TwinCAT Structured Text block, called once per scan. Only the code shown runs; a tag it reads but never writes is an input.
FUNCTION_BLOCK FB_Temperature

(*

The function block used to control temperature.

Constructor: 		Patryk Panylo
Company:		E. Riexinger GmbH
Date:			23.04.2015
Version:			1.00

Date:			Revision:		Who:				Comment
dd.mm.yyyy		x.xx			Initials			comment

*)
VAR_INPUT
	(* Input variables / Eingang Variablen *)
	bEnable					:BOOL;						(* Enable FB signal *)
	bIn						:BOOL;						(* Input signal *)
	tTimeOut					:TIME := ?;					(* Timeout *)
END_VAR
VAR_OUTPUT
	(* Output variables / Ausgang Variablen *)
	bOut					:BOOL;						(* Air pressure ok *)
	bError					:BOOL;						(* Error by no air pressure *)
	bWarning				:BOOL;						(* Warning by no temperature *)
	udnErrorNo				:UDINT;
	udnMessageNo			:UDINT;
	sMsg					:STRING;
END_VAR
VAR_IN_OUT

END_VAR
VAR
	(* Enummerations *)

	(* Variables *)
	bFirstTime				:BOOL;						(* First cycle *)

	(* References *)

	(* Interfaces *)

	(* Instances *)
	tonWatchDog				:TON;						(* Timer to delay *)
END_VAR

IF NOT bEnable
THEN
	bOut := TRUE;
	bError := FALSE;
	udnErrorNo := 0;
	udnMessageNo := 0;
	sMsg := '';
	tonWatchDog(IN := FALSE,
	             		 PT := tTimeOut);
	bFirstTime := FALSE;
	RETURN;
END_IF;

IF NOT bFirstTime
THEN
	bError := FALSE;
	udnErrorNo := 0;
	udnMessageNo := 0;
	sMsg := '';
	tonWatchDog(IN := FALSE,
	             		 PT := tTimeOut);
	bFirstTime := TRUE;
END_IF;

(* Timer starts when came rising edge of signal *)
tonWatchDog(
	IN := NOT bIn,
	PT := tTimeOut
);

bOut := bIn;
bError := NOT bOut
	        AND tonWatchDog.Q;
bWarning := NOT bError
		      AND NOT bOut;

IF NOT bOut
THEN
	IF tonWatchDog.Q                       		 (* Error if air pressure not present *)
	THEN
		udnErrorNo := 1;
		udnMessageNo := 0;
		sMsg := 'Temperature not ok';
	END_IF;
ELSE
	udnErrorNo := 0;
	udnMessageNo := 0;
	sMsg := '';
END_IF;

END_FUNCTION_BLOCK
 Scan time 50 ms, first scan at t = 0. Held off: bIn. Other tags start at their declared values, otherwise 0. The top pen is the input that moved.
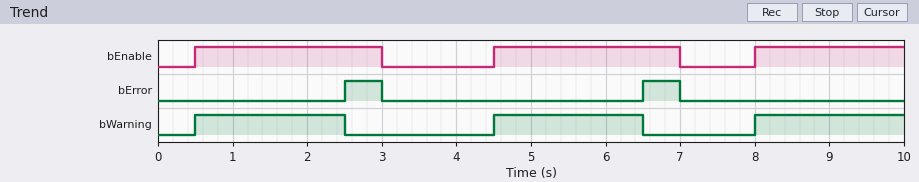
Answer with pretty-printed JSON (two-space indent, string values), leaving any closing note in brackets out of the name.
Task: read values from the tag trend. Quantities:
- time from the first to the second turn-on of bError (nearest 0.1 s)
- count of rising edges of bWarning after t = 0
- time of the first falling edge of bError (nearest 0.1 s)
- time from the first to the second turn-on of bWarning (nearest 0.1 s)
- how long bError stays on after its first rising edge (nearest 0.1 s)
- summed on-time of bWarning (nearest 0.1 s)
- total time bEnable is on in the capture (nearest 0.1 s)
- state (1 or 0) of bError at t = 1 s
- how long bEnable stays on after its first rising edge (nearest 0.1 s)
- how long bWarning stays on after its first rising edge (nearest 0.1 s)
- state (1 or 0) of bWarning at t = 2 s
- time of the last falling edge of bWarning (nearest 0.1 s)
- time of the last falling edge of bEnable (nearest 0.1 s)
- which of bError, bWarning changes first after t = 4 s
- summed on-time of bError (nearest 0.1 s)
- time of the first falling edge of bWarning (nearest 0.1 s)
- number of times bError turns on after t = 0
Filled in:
{
  "time from the first to the second turn-on of bError": "4.0 s",
  "count of rising edges of bWarning after t = 0": "3",
  "time of the first falling edge of bError": "3.0 s",
  "time from the first to the second turn-on of bWarning": "4.0 s",
  "how long bError stays on after its first rising edge": "0.5 s",
  "summed on-time of bWarning": "6.0 s",
  "total time bEnable is on in the capture": "7.0 s",
  "state (1 or 0) of bError at t = 1 s": "0",
  "how long bEnable stays on after its first rising edge": "2.5 s",
  "how long bWarning stays on after its first rising edge": "2.0 s",
  "state (1 or 0) of bWarning at t = 2 s": "1",
  "time of the last falling edge of bWarning": "6.5 s",
  "time of the last falling edge of bEnable": "7.0 s",
  "which of bError, bWarning changes first after t = 4 s": "bWarning",
  "summed on-time of bError": "1.0 s",
  "time of the first falling edge of bWarning": "2.5 s",
  "number of times bError turns on after t = 0": "2"
}
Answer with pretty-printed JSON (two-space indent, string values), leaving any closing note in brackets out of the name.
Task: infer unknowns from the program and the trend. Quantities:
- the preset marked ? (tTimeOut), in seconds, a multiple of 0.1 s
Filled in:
{
  "the preset marked ? (tTimeOut), in seconds, a multiple of 0.1 s": "2.0 s"
}
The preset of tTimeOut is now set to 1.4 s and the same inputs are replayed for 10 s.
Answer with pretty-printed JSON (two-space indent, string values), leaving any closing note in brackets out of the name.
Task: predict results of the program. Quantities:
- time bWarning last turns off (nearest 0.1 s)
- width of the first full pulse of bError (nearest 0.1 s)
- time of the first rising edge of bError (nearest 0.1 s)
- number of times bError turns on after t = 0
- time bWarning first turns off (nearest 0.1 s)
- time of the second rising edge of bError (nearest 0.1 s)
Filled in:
{
  "time bWarning last turns off": "9.4 s",
  "width of the first full pulse of bError": "1.1 s",
  "time of the first rising edge of bError": "1.9 s",
  "number of times bError turns on after t = 0": "3",
  "time bWarning first turns off": "1.9 s",
  "time of the second rising edge of bError": "5.9 s"
}
